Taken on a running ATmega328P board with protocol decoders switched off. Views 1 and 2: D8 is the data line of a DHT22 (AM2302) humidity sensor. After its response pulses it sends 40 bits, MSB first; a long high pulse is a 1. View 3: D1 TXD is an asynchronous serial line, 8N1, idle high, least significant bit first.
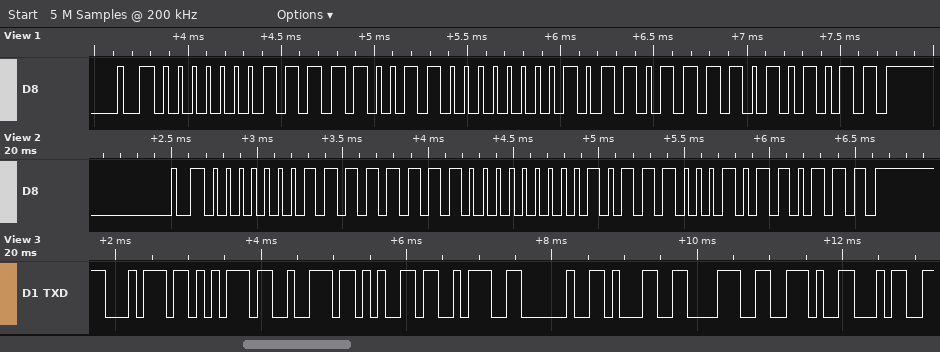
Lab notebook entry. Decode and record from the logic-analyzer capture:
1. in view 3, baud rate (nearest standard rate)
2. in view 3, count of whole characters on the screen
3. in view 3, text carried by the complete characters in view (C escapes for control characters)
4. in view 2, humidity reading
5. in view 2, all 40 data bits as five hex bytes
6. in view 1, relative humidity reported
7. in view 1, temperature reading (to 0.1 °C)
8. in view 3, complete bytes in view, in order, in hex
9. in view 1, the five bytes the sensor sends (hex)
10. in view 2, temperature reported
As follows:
9600 baud
10
"ture: 18.4"
51.0 %
01 FE 00 B8 B7
49.9 %
18.3 °C
74 75 72 65 3A 20 31 38 2E 34
01 F3 00 B7 AB
18.4 °C
